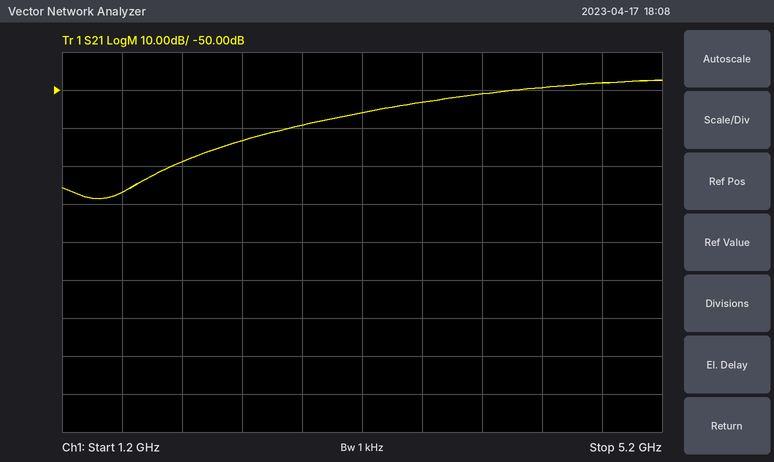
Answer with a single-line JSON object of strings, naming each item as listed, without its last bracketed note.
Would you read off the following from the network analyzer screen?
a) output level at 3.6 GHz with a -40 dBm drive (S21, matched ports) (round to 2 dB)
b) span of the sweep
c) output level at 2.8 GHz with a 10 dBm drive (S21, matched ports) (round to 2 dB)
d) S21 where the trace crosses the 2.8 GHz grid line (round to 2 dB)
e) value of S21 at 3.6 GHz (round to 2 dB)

{"output level at 3.6 GHz with a -40 dBm drive (S21, matched ports)": "-94 dBm", "span of the sweep": "4 GHz", "output level at 2.8 GHz with a 10 dBm drive (S21, matched ports)": "-50 dBm", "S21 where the trace crosses the 2.8 GHz grid line": "-60 dB", "value of S21 at 3.6 GHz": "-54 dB"}
